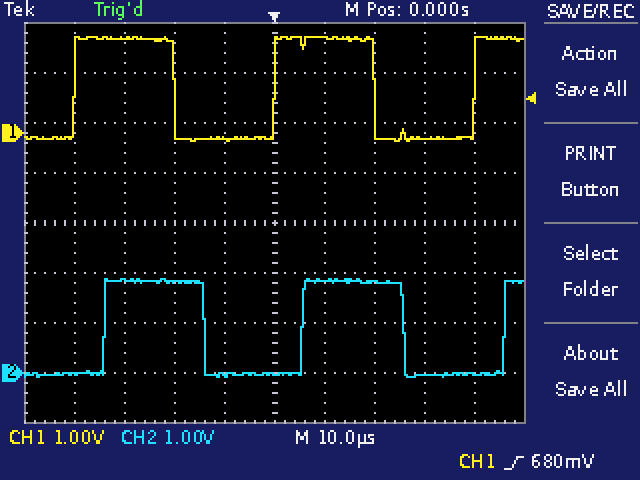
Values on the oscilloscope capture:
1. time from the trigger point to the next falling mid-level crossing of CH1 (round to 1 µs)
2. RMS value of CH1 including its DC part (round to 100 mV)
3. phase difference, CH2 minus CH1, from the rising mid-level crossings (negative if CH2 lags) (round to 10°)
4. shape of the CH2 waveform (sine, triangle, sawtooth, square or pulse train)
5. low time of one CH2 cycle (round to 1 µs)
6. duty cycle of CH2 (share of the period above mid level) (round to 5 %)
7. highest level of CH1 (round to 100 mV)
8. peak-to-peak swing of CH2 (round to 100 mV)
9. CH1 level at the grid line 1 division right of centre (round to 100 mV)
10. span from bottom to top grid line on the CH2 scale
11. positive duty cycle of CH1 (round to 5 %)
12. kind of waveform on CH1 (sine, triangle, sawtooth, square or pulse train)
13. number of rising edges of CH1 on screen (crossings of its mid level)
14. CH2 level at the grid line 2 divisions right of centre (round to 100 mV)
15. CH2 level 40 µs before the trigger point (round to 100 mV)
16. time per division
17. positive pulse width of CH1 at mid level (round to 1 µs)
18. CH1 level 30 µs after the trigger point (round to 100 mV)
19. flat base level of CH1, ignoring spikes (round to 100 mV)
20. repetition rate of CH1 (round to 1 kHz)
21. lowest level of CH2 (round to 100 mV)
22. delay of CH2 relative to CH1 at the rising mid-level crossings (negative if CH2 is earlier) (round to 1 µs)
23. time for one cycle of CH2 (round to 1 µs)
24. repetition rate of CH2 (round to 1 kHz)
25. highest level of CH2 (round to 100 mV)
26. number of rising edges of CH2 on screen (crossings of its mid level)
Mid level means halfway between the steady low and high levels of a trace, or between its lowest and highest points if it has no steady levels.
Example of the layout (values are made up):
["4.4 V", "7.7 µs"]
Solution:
["20 µs", "1.3 V", "-50°", "square", "20 µs", "50 %", "1.9 V", "2.0 V", "1.9 V", "8 V", "50 %", "square", "3", "1.8 V", "0.0 V", "10 µs", "20 µs", "-100 mV", "-100 mV", "25 kHz", "-100 mV", "+6 µs", "40 µs", "25 kHz", "1.9 V", "3"]
